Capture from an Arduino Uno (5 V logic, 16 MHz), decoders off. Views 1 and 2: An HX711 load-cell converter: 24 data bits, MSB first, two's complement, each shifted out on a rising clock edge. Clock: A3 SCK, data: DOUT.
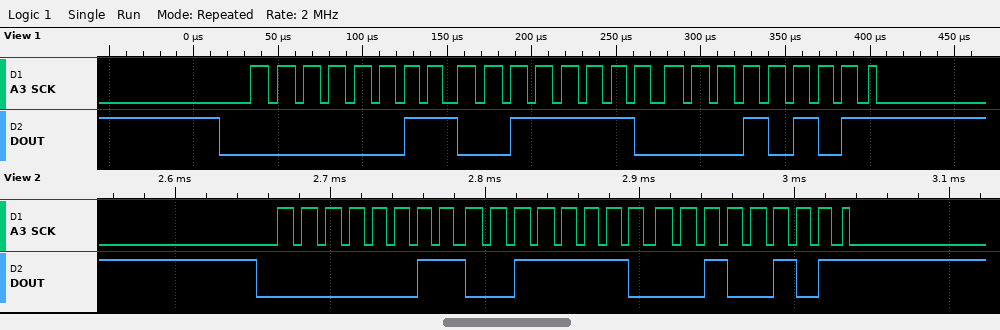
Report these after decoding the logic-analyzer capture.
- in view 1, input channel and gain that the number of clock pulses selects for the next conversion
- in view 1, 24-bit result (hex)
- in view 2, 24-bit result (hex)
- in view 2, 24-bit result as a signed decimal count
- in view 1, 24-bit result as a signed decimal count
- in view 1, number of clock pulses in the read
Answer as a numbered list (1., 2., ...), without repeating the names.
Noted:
1. channel A, gain 128
2. 0x033E15
3. 0x033E25
4. 212517
5. 212501
6. 25
